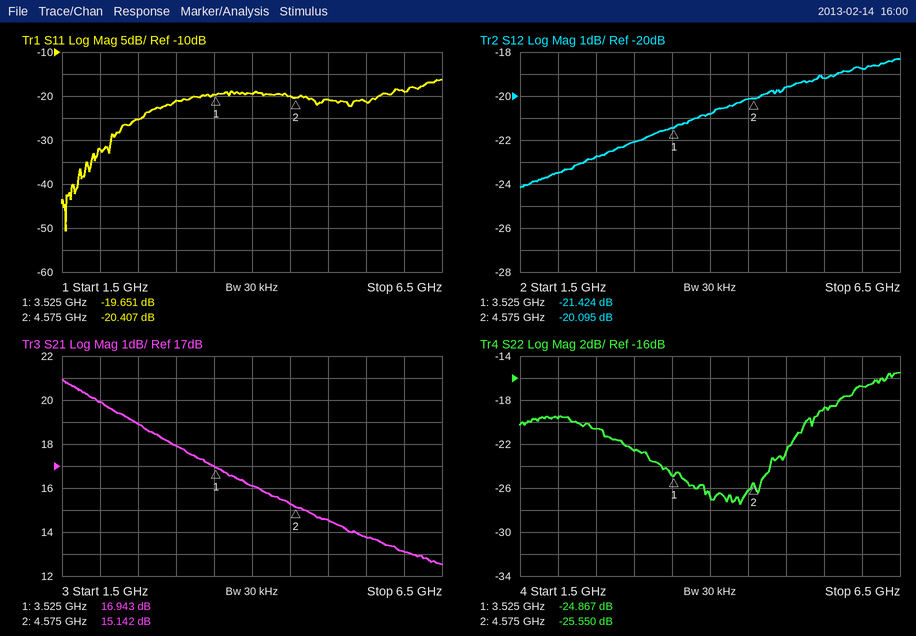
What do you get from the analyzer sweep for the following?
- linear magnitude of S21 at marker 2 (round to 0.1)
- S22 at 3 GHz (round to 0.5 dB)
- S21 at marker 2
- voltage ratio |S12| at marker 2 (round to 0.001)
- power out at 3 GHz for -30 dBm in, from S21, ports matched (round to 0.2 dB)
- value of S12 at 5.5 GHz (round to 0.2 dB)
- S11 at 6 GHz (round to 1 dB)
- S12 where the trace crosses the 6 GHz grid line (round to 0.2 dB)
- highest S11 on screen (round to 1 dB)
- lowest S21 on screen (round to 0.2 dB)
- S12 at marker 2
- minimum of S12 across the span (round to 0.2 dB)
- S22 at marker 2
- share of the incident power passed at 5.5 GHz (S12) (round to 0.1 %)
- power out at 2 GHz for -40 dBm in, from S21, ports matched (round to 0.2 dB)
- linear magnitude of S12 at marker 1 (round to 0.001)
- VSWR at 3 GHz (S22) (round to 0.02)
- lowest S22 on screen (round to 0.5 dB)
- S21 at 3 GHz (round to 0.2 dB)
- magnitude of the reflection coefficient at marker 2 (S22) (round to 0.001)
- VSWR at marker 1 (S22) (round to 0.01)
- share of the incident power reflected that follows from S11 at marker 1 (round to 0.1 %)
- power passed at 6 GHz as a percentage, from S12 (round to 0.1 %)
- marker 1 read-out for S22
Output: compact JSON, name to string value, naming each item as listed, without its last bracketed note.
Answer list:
{"linear magnitude of S21 at marker 2": "5.7", "S22 at 3 GHz": "-22.5 dB", "S21 at marker 2": "15.142 dB", "voltage ratio |S12| at marker 2": "0.099", "power out at 3 GHz for -30 dBm in, from S21, ports matched": "-12.0 dBm", "value of S12 at 5.5 GHz": "-19.2 dB", "S11 at 6 GHz": "-19 dB", "S12 where the trace crosses the 6 GHz grid line": "-18.8 dB", "highest S11 on screen": "-16 dB", "lowest S21 on screen": "12.6 dB", "S12 at marker 2": "-20.095 dB", "minimum of S12 across the span": "-24.2 dB", "S22 at marker 2": "-25.550 dB", "share of the incident power passed at 5.5 GHz (S12)": "1.2 %", "power out at 2 GHz for -40 dBm in, from S21, ports matched": "-20.0 dBm", "linear magnitude of S12 at marker 1": "0.085", "VSWR at 3 GHz (S22)": "1.16", "lowest S22 on screen": "-27.5 dB", "S21 at 3 GHz": "18.0 dB", "magnitude of the reflection coefficient at marker 2 (S22)": "0.053", "VSWR at marker 1 (S22)": "1.12", "share of the incident power reflected that follows from S11 at marker 1": "1.1 %", "power passed at 6 GHz as a percentage, from S12": "1.3 %", "marker 1 read-out for S22": "-24.867 dB"}
